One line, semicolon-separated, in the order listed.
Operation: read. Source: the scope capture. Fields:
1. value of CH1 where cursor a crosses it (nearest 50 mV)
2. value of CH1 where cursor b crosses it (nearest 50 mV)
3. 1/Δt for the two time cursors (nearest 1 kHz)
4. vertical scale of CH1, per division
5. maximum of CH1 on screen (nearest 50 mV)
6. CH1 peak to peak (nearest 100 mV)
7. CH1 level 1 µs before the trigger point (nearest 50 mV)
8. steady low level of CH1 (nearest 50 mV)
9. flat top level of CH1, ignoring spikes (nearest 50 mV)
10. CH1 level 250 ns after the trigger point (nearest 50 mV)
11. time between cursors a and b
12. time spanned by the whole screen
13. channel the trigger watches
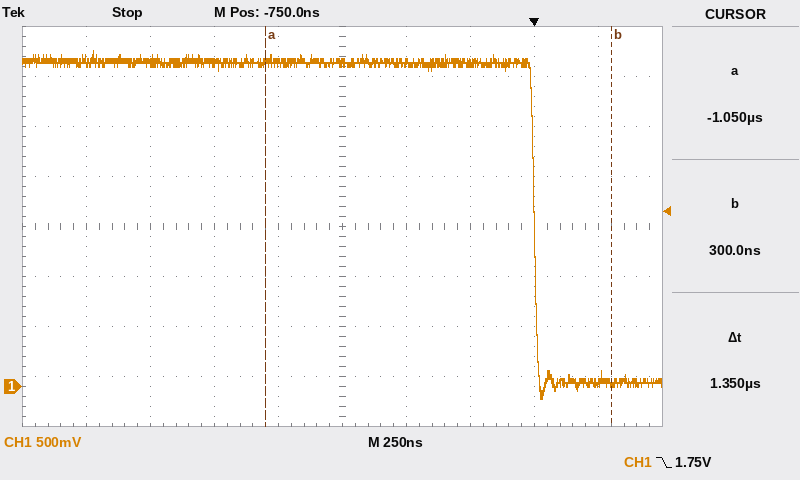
3.25 V; 50 mV; 741 kHz; 500 mV; 3.35 V; 3.50 V; 3.25 V; 50 mV; 3.25 V; 50 mV; 1.35 µs; 2.5 µs; CH1
